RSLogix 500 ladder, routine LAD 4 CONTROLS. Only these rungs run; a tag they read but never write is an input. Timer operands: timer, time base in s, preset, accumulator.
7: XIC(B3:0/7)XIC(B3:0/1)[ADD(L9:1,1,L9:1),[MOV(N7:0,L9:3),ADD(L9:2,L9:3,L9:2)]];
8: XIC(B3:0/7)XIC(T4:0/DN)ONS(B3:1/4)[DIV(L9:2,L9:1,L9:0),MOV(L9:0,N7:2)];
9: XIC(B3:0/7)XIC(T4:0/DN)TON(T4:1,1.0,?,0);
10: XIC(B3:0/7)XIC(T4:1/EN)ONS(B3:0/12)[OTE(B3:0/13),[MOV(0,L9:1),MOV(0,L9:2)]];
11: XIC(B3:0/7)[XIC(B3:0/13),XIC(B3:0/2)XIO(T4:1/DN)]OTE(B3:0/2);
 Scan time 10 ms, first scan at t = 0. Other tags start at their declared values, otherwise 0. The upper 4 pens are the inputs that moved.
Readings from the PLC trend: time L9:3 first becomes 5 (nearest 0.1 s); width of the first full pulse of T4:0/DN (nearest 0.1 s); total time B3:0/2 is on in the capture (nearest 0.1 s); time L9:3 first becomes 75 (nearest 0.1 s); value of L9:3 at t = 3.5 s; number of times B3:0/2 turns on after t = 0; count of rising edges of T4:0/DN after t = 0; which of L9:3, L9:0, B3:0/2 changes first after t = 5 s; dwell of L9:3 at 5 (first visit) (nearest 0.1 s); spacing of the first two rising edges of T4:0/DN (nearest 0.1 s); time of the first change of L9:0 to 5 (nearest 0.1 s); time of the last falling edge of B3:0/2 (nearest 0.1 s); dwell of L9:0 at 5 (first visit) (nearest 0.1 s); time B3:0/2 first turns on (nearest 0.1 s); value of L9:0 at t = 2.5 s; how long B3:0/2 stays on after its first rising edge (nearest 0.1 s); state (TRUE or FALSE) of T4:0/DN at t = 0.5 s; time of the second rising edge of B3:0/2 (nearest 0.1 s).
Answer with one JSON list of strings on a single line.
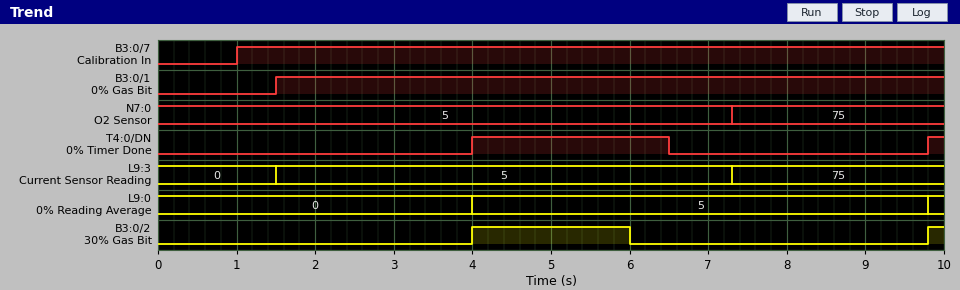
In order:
["1.5 s", "2.5 s", "2.2 s", "7.3 s", "5", "2", "2", "B3:0/2", "5.8 s", "5.8 s", "4.0 s", "6.0 s", "5.8 s", "4.0 s", "0", "2.0 s", "FALSE", "9.8 s"]
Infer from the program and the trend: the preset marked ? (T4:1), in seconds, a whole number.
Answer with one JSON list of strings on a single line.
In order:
["2 s"]
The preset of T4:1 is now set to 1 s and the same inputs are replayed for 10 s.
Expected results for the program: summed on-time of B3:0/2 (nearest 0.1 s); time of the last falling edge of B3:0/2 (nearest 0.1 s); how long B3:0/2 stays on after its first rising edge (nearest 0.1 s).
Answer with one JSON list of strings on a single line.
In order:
["1.2 s", "5.0 s", "1.0 s"]
